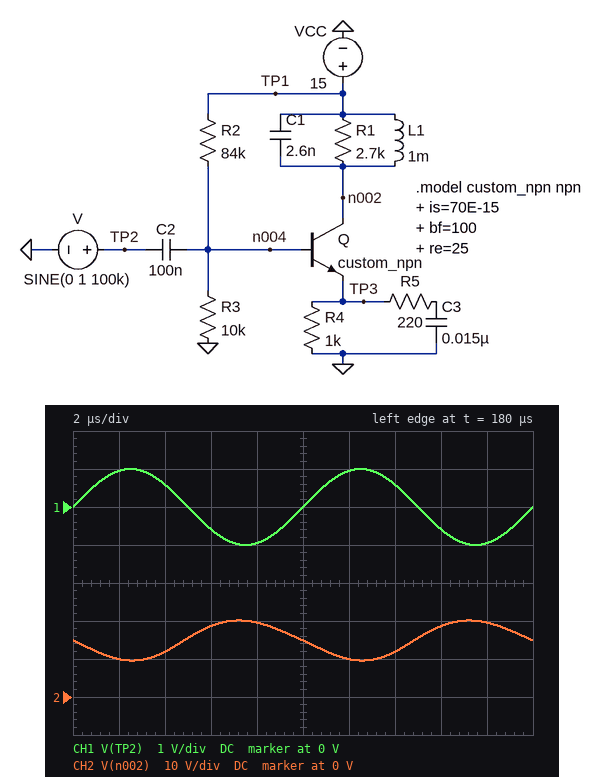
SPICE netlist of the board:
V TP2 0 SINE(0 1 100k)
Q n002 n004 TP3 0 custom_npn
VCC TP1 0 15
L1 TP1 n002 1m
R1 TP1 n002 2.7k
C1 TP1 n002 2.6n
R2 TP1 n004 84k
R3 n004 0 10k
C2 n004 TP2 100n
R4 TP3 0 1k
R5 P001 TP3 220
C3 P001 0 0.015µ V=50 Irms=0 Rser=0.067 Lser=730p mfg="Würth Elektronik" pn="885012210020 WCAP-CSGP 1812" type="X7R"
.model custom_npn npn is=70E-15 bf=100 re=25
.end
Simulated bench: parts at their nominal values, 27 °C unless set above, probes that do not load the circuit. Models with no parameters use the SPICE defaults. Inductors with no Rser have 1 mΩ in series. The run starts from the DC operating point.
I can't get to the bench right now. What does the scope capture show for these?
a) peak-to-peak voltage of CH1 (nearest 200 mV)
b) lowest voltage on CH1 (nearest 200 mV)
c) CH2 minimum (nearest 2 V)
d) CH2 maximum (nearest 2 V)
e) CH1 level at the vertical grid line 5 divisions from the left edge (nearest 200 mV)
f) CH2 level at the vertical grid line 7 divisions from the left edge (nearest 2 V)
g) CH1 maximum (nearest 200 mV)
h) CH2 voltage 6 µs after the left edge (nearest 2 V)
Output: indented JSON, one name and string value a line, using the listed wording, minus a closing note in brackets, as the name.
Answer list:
{
  "peak-to-peak voltage of CH1": "2.0 V",
  "lowest voltage on CH1": "-1.0 V",
  "CH2 minimum": "10 V",
  "CH2 maximum": "20 V",
  "CH1 level at the vertical grid line 5 divisions from the left edge": "0 V",
  "CH2 level at the vertical grid line 7 divisions from the left edge": "12 V",
  "CH1 maximum": "1.0 V",
  "CH2 voltage 6 µs after the left edge": "18 V"
}
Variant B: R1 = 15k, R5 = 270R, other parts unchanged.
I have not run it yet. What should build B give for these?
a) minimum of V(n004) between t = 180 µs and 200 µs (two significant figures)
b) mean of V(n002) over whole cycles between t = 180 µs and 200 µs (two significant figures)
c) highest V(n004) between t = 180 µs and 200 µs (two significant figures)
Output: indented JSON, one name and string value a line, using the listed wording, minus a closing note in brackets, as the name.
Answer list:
{
  "minimum of V(n004) between t = 180 µs and 200 µs": "110 mV",
  "mean of V(n002) over whole cycles between t = 180 µs and 200 µs": "15 V",
  "highest V(n004) between t = 180 µs and 200 µs": "2.1 V"
}
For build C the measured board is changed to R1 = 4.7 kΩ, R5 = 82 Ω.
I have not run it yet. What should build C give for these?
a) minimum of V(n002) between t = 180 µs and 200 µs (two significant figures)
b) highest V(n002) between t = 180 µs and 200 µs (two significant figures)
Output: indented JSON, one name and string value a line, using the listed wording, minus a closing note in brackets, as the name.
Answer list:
{
  "minimum of V(n002) between t = 180 µs and 200 µs": "4.0 V",
  "highest V(n002) between t = 180 µs and 200 µs": "25 V"
}
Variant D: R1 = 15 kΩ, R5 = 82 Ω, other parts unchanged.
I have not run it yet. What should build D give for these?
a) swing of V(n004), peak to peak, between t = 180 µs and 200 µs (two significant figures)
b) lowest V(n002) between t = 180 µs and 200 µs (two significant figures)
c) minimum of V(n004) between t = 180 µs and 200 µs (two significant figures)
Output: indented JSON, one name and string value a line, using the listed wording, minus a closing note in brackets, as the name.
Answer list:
{
  "swing of V(n004), peak to peak, between t = 180 µs and 200 µs": "2.0 V",
  "lowest V(n002) between t = 180 µs and 200 µs": "1.3 V",
  "minimum of V(n004) between t = 180 µs and 200 µs": "-79 mV"
}
